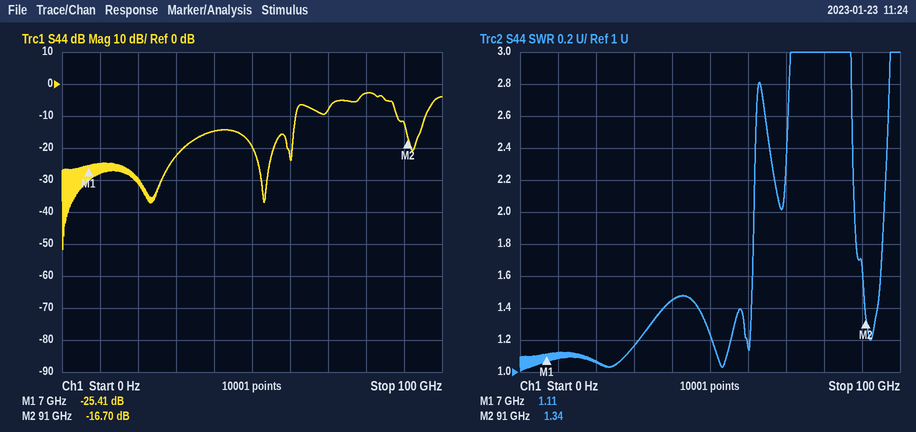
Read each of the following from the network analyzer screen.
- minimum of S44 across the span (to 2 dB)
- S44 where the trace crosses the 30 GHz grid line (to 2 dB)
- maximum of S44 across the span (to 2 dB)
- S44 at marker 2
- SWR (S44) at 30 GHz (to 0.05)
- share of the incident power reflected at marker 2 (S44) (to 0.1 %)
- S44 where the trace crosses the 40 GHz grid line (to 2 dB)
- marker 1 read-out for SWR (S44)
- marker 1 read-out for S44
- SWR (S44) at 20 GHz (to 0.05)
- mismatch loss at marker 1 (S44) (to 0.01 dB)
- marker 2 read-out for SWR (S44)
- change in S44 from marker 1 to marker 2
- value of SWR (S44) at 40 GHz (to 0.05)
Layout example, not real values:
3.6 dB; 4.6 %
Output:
-52 dB; -22 dB; -2 dB; -16.70 dB; 1.15; 2.1 %; -14 dB; 1.11; -25.41 dB; 1.05; 0.01 dB; 1.34; 8.71 dB; 1.45
